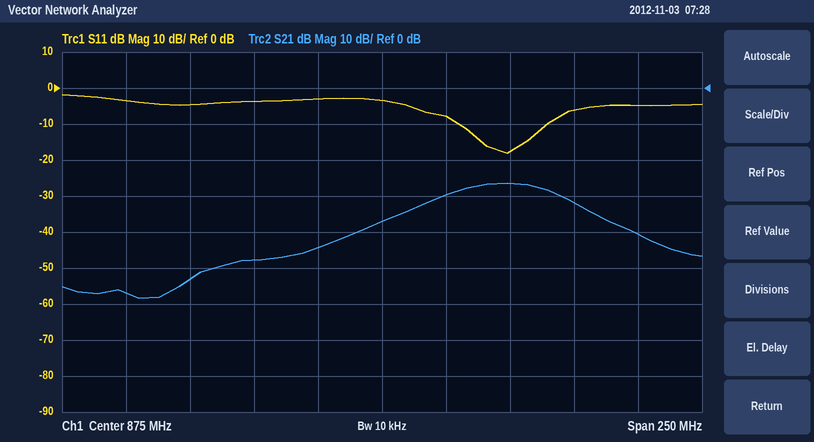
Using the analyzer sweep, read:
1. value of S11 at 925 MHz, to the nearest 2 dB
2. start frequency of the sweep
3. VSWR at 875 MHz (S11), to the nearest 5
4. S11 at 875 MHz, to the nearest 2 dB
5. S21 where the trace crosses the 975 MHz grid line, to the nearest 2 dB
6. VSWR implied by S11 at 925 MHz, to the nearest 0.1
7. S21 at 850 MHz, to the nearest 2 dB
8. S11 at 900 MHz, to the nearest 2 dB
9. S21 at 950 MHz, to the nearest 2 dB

-18 dB
750 MHz
5
-4 dB
-40 dB
1.3
-44 dB
-8 dB
-32 dB
